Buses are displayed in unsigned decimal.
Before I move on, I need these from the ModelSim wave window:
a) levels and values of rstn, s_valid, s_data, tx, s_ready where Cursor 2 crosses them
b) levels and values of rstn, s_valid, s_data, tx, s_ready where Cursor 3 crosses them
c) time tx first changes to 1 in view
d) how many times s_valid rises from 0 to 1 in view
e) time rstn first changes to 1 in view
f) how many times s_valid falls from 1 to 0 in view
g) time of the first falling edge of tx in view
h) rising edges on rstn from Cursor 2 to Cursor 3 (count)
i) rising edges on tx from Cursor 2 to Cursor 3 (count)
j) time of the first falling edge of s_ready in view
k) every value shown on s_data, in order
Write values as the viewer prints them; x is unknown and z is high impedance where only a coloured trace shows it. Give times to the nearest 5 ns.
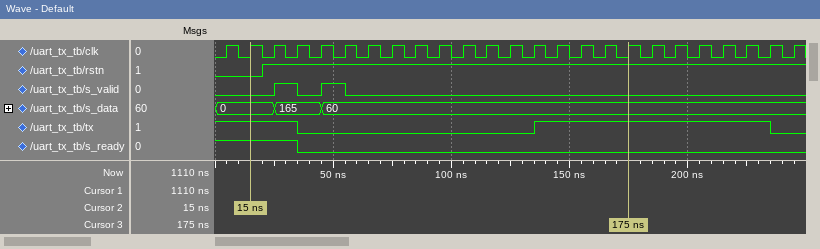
rstn=0, s_valid=0, s_data=0, tx=1, s_ready=1
rstn=1, s_valid=0, s_data=60, tx=1, s_ready=0
135 ns
2
20 ns
2
35 ns
1
1
35 ns
0, 165, 60
